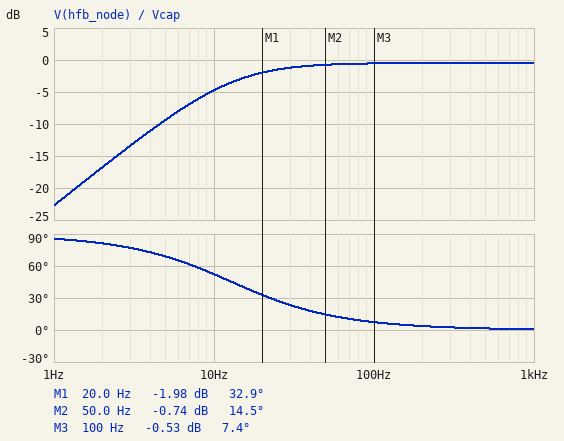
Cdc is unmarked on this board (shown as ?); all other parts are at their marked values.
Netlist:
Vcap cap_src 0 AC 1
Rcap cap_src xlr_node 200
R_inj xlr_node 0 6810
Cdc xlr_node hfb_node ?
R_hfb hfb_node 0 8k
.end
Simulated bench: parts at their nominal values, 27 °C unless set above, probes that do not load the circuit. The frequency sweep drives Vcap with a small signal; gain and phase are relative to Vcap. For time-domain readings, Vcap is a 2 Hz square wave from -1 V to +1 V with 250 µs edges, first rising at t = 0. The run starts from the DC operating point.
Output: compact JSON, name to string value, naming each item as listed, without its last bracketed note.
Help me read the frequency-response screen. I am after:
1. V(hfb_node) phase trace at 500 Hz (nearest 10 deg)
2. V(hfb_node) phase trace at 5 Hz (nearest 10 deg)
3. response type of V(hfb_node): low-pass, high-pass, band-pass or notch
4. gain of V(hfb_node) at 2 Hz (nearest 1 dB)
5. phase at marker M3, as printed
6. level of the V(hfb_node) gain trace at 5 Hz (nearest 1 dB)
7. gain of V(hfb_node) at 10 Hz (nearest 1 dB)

{"V(hfb_node) phase trace at 500 Hz": "0 deg", "V(hfb_node) phase trace at 5 Hz": "70 deg", "response type of V(hfb_node): low-pass, high-pass, band-pass or notch": "high-pass", "gain of V(hfb_node) at 2 Hz": "-17 dB", "phase at marker M3, as printed": "7.4 deg", "level of the V(hfb_node) gain trace at 5 Hz": "-9 dB", "gain of V(hfb_node) at 10 Hz": "-5 dB"}
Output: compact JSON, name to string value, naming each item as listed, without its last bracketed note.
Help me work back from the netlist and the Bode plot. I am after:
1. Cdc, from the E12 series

{"Cdc, from the E12 series": "1.5 µF"}
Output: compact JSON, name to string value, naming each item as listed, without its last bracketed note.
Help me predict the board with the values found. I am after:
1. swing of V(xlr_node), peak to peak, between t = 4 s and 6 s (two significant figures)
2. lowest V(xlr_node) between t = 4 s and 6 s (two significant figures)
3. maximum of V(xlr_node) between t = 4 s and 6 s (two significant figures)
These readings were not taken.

{"swing of V(xlr_node), peak to peak, between t = 4 s and 6 s": "1.9 V", "lowest V(xlr_node) between t = 4 s and 6 s": "-970 mV", "maximum of V(xlr_node) between t = 4 s and 6 s": "970 mV"}
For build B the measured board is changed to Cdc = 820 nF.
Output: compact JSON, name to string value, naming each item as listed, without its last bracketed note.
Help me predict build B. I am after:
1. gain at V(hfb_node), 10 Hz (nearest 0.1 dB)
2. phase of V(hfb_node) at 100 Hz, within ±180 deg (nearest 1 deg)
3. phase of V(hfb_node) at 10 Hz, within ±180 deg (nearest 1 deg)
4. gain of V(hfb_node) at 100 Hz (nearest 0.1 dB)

{"gain at V(hfb_node), 10 Hz": "-8.7 dB", "phase of V(hfb_node) at 100 Hz, within ±180 deg": "13 deg", "phase of V(hfb_node) at 10 Hz, within ±180 deg": "67 deg", "gain of V(hfb_node) at 100 Hz": "-0.7 dB"}
